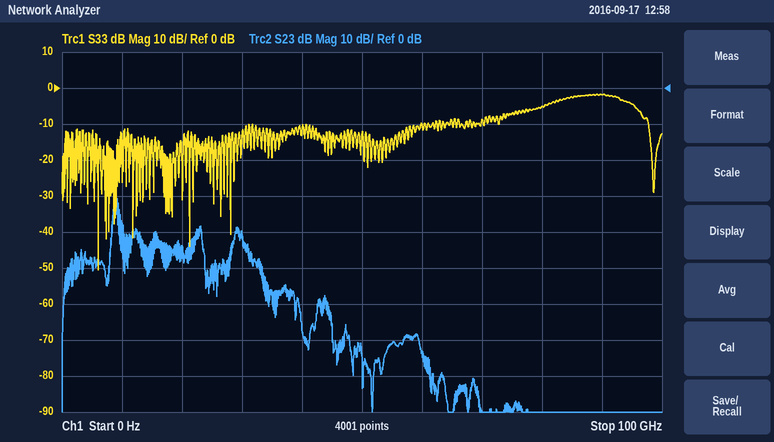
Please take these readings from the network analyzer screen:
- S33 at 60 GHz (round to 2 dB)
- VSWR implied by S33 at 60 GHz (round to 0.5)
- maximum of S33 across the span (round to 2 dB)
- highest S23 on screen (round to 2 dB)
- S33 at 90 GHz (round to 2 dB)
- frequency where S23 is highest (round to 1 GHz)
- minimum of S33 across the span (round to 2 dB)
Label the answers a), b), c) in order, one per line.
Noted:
a) -10 dB
b) 2.0
c) -2 dB
d) -30 dB
e) -2 dB
f) 9 GHz
g) -50 dB
